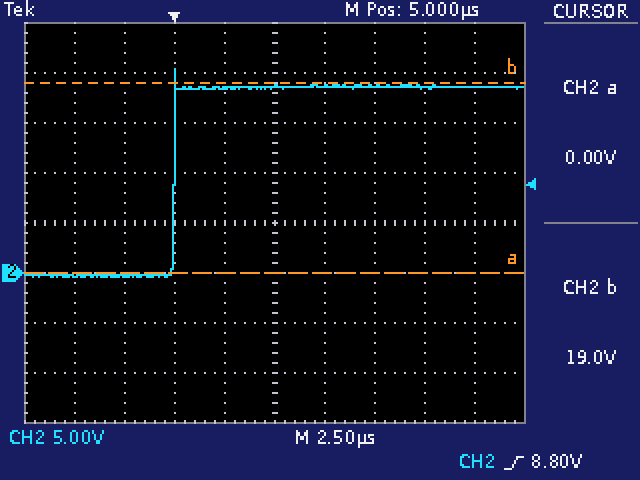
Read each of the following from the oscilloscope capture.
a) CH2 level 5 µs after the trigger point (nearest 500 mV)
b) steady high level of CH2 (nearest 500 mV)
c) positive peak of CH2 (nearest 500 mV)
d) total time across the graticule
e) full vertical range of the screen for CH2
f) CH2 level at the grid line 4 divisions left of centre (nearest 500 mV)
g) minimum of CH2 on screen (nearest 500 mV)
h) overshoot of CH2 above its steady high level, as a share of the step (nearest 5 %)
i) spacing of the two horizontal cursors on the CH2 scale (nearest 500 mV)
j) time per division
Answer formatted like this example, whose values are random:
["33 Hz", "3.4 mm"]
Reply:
["18.5 V", "18.5 V", "20.5 V", "25 µs", "40 V", "-500 mV", "-500 mV", "10 %", "19.0 V", "2.5 µs"]
